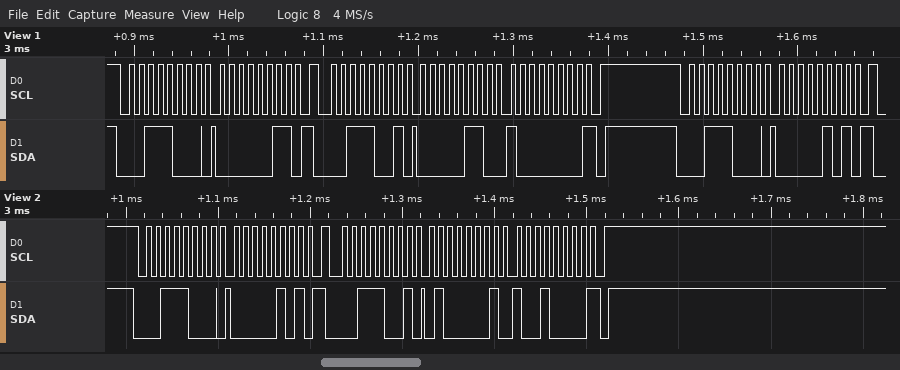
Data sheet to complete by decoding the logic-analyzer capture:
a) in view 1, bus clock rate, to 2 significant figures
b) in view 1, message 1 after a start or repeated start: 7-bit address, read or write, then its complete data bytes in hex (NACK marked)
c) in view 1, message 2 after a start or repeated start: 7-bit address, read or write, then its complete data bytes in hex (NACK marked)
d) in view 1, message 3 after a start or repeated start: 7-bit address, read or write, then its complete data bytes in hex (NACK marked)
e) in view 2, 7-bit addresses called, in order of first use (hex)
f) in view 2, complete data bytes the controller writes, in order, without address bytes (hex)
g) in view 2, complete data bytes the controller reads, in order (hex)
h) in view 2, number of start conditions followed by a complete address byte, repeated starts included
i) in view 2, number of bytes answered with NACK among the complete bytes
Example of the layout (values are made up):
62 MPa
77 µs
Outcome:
100 kHz
0x1C write: 03
0x1C read: 06 80 NACK
0x1C write: 05
0x1C
05
41 90
2
1
